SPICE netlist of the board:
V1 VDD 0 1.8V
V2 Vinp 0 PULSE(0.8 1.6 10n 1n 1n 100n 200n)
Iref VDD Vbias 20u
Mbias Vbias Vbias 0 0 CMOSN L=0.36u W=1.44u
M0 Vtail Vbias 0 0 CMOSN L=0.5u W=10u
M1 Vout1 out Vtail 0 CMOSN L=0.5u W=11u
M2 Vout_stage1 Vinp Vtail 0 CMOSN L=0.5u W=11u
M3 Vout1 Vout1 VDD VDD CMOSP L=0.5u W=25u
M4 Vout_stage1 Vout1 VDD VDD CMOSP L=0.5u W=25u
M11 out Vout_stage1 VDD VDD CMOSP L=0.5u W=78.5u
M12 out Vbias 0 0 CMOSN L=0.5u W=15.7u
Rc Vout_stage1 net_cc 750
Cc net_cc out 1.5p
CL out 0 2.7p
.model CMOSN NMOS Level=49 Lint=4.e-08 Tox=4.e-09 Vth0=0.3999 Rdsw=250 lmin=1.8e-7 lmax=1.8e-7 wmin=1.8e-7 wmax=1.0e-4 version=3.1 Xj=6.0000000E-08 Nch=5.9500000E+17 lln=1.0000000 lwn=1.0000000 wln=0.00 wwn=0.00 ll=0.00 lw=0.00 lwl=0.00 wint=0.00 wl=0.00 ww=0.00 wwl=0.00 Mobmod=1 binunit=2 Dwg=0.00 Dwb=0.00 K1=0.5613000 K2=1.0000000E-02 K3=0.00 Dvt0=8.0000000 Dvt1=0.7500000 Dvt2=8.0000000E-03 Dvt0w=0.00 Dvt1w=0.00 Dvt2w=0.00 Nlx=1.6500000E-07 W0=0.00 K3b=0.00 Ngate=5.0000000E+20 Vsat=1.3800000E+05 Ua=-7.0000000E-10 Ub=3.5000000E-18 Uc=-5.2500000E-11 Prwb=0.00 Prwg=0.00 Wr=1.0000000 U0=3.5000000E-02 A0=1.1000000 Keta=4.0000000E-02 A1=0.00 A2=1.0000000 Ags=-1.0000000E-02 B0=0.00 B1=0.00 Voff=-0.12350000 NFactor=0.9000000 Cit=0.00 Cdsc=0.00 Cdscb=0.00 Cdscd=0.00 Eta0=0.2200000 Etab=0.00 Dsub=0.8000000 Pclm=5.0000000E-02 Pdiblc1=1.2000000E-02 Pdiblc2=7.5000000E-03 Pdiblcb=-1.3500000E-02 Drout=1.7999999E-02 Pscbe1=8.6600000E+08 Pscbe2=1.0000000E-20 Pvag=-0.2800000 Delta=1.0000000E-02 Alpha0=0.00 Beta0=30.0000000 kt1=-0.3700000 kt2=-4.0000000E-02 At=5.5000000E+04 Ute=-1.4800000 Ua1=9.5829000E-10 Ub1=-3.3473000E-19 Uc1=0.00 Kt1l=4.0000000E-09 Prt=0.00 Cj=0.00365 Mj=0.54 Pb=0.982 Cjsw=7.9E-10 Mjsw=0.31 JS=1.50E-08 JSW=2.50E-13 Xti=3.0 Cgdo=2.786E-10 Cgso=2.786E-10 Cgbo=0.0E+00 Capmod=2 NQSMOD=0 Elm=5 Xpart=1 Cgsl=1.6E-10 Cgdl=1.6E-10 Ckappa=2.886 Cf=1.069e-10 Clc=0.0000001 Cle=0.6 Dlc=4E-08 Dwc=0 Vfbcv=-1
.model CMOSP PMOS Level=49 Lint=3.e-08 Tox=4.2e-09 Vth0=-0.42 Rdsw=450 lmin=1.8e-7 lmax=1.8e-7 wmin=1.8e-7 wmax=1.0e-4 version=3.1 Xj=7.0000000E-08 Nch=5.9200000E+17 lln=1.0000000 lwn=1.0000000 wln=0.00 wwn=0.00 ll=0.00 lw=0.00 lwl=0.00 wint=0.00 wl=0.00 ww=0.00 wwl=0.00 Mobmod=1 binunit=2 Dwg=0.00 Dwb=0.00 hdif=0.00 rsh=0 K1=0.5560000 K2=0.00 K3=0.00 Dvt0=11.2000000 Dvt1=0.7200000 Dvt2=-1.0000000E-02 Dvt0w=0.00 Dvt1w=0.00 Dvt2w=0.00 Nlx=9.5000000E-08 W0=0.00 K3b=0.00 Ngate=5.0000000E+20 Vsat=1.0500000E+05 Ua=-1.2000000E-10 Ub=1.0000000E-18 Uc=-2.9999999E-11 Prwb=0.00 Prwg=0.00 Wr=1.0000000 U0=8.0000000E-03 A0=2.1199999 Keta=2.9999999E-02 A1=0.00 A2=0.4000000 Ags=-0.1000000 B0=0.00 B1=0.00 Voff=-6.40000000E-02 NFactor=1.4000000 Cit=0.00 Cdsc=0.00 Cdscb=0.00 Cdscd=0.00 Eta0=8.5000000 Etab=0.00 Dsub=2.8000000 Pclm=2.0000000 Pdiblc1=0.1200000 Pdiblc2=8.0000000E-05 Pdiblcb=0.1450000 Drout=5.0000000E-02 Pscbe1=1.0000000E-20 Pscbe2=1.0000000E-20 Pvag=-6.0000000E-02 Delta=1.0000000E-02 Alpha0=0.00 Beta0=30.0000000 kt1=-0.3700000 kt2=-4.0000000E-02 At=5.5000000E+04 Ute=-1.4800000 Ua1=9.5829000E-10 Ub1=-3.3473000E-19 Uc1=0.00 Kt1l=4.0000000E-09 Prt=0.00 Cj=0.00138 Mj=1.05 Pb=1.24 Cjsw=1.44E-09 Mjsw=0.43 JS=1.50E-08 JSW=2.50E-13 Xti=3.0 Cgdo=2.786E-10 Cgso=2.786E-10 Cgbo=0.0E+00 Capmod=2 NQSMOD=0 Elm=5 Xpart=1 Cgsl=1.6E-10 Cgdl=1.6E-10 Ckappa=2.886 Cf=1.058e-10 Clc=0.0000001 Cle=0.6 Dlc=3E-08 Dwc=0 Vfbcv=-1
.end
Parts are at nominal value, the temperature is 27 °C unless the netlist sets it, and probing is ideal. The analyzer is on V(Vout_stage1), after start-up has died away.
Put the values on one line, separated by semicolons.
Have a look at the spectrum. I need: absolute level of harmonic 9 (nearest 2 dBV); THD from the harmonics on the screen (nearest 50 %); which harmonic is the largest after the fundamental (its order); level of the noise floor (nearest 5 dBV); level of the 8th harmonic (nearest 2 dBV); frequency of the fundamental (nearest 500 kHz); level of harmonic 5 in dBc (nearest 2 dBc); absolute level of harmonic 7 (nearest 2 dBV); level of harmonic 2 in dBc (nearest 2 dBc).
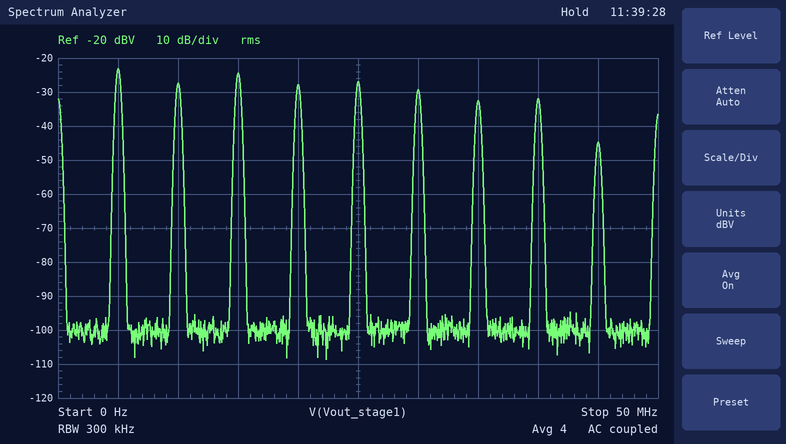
-44 dBV; 150 %; 3; -100 dBV; -32 dBV; 5.0 MHz; -4 dBc; -32 dBV; -4 dBc
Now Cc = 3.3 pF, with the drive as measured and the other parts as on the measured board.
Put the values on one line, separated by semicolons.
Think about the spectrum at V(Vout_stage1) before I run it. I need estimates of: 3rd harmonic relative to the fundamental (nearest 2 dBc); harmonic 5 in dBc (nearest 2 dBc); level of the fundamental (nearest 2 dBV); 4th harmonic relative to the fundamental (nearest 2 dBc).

-2 dBc; -8 dBc; -26 dBV; -12 dBc
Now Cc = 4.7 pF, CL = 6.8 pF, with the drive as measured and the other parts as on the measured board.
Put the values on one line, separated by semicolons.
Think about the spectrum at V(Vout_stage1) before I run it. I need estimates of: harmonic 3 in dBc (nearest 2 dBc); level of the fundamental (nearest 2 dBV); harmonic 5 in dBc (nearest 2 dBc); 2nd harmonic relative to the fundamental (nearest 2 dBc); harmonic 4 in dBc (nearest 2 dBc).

-10 dBc; -18 dBV; -14 dBc; -6 dBc; -14 dBc
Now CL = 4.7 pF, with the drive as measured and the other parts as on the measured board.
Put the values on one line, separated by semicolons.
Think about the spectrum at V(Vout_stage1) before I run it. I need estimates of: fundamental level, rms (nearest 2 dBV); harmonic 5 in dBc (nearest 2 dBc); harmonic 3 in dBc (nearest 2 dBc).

-18 dBV; -10 dBc; -2 dBc
